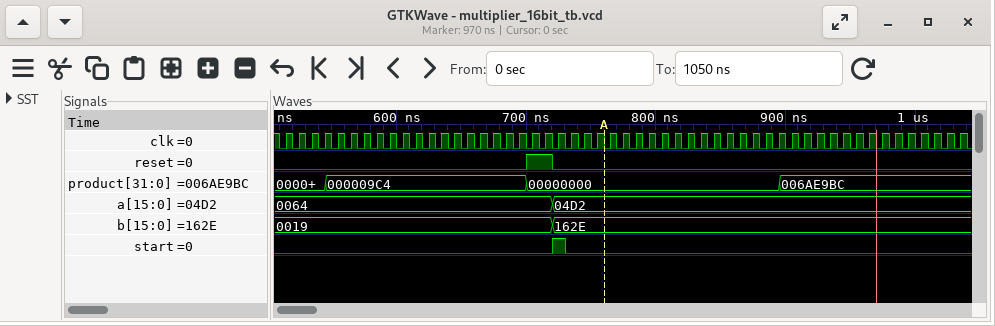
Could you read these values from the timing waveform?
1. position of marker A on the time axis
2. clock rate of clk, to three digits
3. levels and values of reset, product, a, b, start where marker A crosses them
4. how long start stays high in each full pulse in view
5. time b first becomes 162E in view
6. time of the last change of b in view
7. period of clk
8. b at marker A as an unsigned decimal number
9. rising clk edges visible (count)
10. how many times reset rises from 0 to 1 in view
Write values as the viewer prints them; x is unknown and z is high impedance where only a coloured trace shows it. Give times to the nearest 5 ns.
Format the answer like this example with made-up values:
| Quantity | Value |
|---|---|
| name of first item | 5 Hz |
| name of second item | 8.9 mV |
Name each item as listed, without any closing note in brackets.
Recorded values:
| Quantity | Value |
|---|---|
| position of marker A on the time axis | 760 ns |
| clock rate of clk, to three digits | 100 MHz |
| levels and values of reset, product, a, b, start where marker A crosses them | reset=0, product=00000000, a=04D2, b=162E, start=0 |
| how long start stays high in each full pulse in view | 10 ns |
| time b first becomes 162E in view | 720 ns |
| time of the last change of b in view | 720 ns |
| period of clk | 10 ns |
| b at marker A as an unsigned decimal number | 5678 |
| rising clk edges visible | 53 |
| how many times reset rises from 0 to 1 in view | 1 |
